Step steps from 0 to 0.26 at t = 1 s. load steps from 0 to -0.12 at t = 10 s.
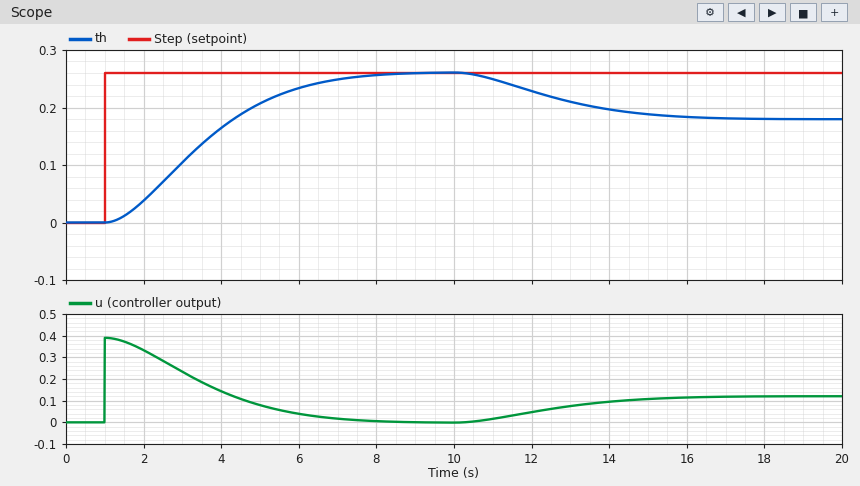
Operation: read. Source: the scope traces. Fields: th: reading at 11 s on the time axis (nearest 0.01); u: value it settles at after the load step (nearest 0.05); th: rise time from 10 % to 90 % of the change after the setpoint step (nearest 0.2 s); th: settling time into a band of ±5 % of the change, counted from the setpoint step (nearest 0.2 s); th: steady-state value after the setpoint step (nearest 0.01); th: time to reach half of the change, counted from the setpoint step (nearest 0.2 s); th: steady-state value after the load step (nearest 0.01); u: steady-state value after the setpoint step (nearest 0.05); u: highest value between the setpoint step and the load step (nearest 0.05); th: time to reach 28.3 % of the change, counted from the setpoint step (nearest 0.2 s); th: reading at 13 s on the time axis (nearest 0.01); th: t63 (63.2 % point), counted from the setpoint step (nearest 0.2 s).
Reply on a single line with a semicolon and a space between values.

0.25; 0.10; 4.2 s; 5.8 s; 0.26; 2.4 s; 0.18; 0.00; 0.40; 1.6 s; 0.21; 3.0 s
